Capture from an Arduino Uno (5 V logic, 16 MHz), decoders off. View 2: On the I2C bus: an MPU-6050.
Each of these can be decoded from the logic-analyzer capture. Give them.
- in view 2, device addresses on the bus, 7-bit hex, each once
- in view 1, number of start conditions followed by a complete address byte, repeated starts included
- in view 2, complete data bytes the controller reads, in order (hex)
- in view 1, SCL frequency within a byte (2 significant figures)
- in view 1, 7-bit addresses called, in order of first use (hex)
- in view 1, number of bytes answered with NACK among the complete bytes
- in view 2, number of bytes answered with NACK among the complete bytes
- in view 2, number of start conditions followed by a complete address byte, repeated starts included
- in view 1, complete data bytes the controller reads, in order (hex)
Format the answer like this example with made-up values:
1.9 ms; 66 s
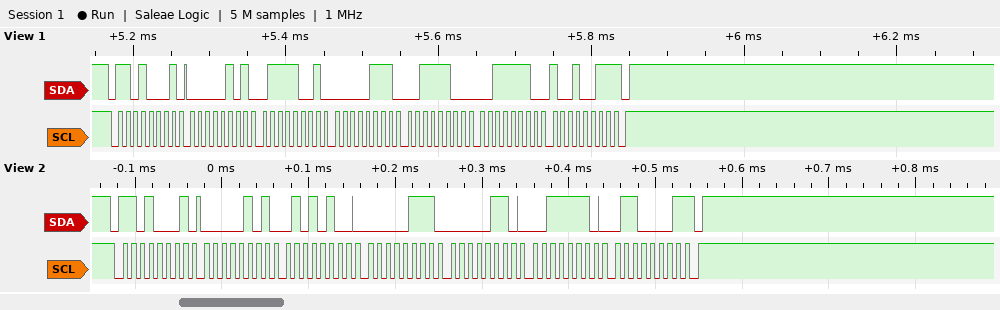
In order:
0x68; 1; 05 54 07 06 3E 61; 100 kHz; 0x68; 1; 1; 1; 05 79 07 3C 3E 93
